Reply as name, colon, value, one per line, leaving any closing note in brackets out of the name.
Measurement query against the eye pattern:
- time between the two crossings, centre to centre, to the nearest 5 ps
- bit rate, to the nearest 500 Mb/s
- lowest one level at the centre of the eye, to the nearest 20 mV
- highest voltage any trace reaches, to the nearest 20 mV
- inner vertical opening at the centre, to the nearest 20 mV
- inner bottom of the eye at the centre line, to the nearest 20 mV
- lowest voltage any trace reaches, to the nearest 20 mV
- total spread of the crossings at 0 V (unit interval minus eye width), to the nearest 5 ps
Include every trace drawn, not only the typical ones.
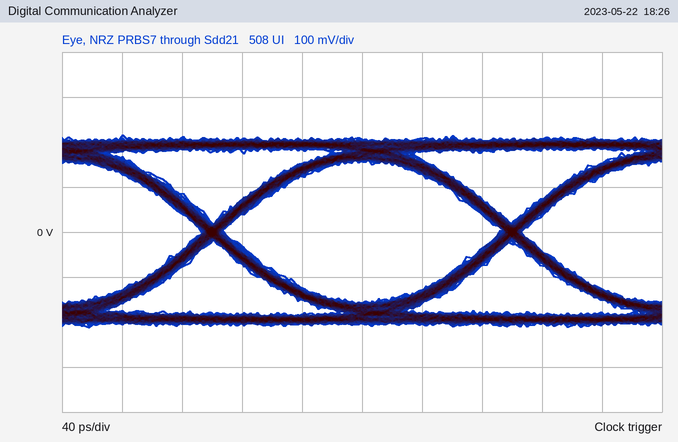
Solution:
time between the two crossings, centre to centre, to the nearest 5 ps: 200 ps
bit rate, to the nearest 500 Mb/s: 5.0 Gb/s
lowest one level at the centre of the eye, to the nearest 20 mV: 160 mV
highest voltage any trace reaches, to the nearest 20 mV: 220 mV
inner vertical opening at the centre, to the nearest 20 mV: 320 mV
inner bottom of the eye at the centre line, to the nearest 20 mV: -160 mV
lowest voltage any trace reaches, to the nearest 20 mV: -220 mV
total spread of the crossings at 0 V (unit interval minus eye width), to the nearest 5 ps: 15 ps
